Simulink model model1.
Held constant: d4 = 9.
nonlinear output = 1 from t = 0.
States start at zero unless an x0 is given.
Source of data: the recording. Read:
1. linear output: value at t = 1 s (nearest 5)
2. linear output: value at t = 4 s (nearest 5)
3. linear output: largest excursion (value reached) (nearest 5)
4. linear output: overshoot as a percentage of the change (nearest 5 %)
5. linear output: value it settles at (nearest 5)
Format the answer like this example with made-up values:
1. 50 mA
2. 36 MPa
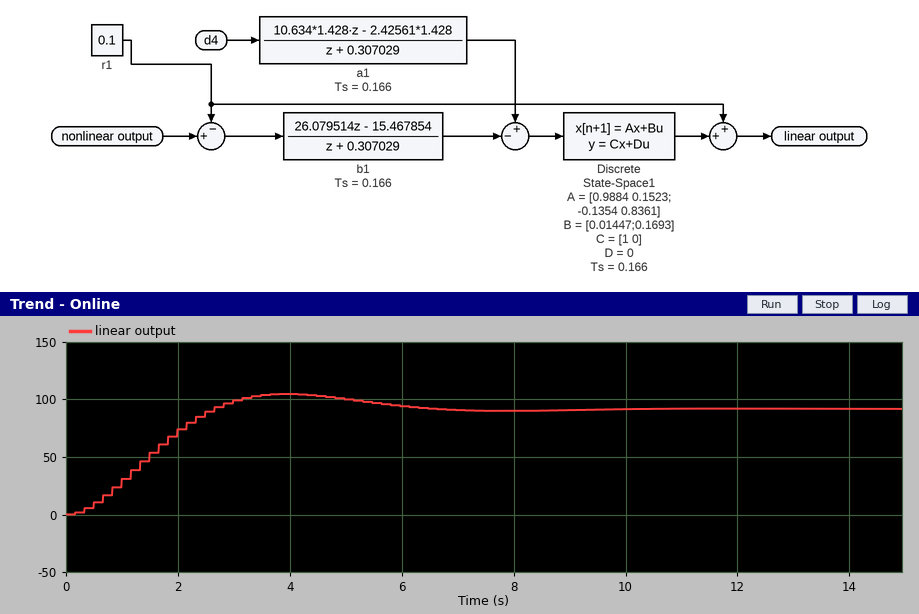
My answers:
1. 30
2. 105
3. 105
4. 15 %
5. 90
